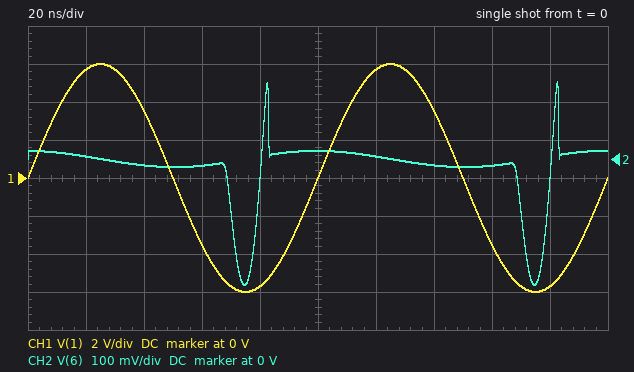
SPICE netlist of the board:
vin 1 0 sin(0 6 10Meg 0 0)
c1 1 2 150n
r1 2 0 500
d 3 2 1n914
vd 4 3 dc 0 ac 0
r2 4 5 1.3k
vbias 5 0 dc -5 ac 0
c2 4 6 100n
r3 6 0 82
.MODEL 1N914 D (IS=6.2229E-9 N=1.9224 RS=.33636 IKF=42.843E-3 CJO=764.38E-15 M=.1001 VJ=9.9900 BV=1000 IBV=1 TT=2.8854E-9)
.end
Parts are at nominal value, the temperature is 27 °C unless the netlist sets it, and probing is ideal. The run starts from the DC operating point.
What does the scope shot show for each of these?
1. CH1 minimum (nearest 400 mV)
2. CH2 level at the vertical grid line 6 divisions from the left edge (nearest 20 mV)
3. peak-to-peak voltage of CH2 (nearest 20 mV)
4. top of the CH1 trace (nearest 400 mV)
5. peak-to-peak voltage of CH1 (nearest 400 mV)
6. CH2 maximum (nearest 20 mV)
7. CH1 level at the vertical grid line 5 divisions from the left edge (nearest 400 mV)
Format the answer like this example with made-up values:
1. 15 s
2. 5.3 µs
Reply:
1. -6.0 V
2. 0 V
3. 540 mV
4. 6.0 V
5. 12.0 V
6. 200 mV
7. 0 V
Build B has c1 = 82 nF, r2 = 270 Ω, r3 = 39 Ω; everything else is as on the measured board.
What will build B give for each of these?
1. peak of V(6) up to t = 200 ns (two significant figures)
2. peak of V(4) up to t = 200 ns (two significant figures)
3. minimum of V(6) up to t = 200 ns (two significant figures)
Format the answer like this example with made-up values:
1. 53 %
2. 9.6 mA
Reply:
1. 180 mV
2. -4.8 V
3. -290 mV
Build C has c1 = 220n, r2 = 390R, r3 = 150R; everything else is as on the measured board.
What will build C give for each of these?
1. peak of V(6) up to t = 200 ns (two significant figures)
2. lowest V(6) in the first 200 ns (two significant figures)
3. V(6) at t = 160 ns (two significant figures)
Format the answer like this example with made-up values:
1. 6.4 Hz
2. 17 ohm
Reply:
1. 210 mV
2. -350 mV
3. -25 mV
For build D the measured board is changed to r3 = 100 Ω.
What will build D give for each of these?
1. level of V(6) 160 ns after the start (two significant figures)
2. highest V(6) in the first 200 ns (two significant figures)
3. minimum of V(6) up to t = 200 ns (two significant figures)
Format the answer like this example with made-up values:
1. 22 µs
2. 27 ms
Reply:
1. -21 mV
2. 210 mV
3. -340 mV
